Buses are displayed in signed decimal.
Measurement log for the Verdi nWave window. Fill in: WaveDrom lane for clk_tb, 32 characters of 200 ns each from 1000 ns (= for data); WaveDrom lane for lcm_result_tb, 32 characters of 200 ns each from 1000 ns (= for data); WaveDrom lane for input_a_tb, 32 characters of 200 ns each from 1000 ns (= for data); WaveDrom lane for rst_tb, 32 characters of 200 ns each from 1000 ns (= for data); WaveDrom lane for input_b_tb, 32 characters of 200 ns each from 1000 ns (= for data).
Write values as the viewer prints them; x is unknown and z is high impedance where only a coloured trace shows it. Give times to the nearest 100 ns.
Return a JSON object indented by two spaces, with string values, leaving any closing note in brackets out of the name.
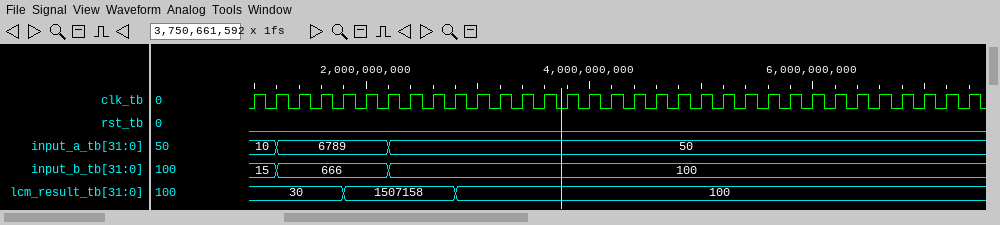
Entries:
{
  "WaveDrom lane for clk_tb, 32 characters of 200 ns each from 1000 ns": "{name: 'clk_tb', wave: 'p...............................'}",
  "WaveDrom lane for lcm_result_tb, 32 characters of 200 ns each from 1000 ns": "{name: 'lcm_result_tb', wave: '=...=....=......................', data: '30 1507158 100'}",
  "WaveDrom lane for input_a_tb, 32 characters of 200 ns each from 1000 ns": "{name: 'input_a_tb', wave: '==....=.........................', data: '10 6789 50'}",
  "WaveDrom lane for rst_tb, 32 characters of 200 ns each from 1000 ns": "{name: 'rst_tb', wave: '0...............................'}",
  "WaveDrom lane for input_b_tb, 32 characters of 200 ns each from 1000 ns": "{name: 'input_b_tb', wave: '==....=.........................', data: '15 666 100'}"
}
